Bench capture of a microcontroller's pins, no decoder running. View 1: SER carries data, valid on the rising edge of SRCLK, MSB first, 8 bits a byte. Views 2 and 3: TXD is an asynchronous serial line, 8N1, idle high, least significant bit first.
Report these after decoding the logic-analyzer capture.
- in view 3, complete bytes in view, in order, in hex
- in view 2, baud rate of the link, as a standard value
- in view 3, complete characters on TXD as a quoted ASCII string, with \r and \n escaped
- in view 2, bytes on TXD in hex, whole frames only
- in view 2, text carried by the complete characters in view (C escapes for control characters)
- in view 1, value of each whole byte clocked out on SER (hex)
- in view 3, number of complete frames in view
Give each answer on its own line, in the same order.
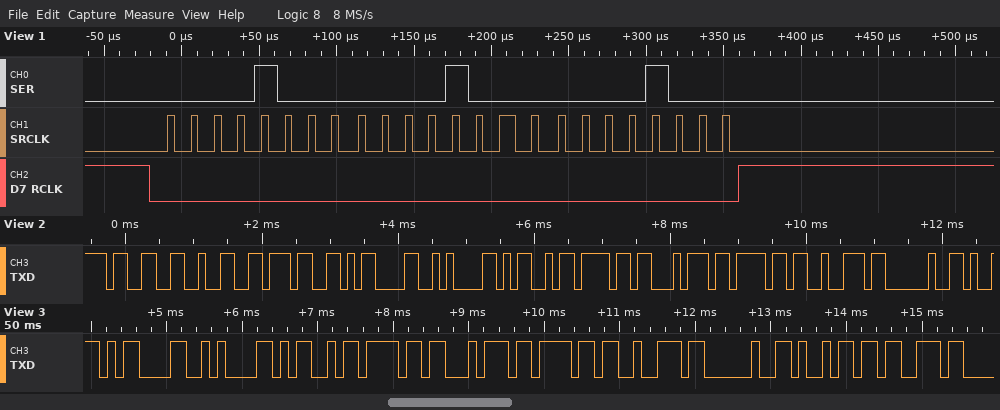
0D 0A 4D 6F 74 6F 72 20 69 73
9600 baud
"\r\nMotor is"
33 32 37 0D 0A 4D 6F 74 6F 72 20
"327\r\nMotor "
08 08 08
10
